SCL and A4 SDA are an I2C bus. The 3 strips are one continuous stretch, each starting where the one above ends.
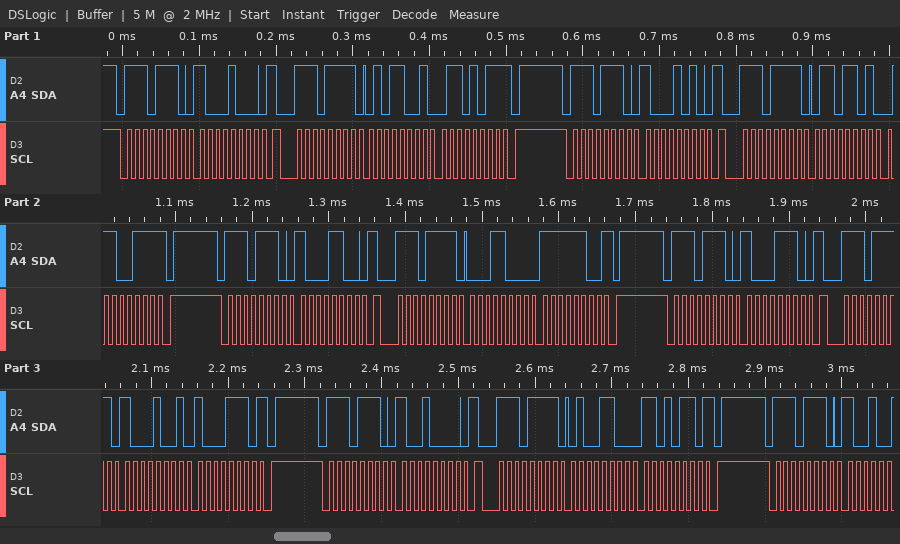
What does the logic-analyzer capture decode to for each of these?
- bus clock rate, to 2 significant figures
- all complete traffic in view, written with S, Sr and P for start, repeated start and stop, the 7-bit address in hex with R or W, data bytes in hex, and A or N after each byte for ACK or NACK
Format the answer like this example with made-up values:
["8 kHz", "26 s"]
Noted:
["100 kHz", "S 77W A 88 A Sr 77R A 59 A 6B N P S 77W A 8A A Sr 77R A 6D A 67 N P S 77W A 8C A Sr 77R A 18 A FC N P S 77W A 8E A Sr 77R A 89 A 8E N P S 77W A 90 A Sr 77R A 4C A D6 N P S 77W A"]
